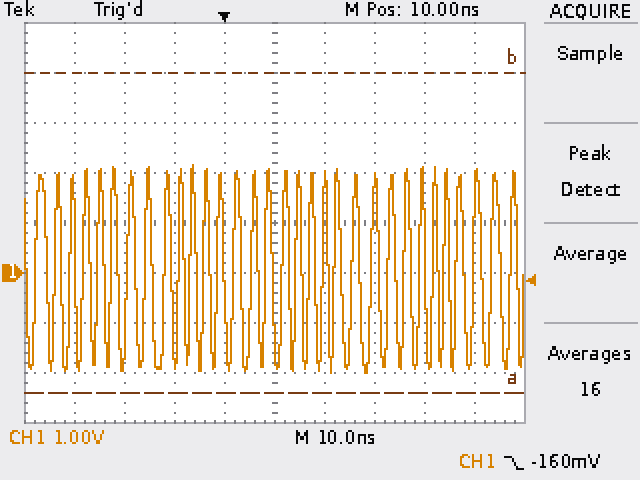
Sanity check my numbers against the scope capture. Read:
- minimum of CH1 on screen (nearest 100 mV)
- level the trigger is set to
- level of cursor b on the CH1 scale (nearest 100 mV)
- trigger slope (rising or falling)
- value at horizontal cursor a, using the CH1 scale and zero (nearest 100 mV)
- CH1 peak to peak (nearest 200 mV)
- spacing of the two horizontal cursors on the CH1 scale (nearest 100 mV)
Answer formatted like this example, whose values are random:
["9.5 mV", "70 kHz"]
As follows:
["-2.0 V", "-160 mV", "4.0 V", "falling", "-2.4 V", "4.2 V", "6.4 V"]
